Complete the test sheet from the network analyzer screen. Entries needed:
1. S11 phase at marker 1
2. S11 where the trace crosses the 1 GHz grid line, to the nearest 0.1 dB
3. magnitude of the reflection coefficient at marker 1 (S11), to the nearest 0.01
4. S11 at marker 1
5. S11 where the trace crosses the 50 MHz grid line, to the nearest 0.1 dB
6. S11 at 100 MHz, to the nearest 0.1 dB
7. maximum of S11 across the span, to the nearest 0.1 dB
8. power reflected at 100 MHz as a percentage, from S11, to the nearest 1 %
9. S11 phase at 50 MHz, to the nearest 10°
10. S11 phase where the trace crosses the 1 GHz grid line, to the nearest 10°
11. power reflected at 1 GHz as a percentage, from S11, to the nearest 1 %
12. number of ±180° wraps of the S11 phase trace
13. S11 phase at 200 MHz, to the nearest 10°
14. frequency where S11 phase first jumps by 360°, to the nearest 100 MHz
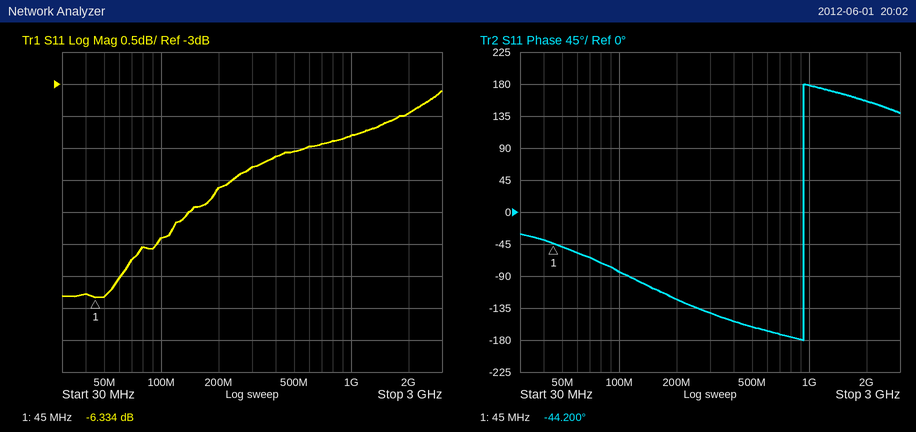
-44.200°
-3.8 dB
0.48
-6.334 dB
-6.3 dB
-5.4 dB
-3.1 dB
29 %
-50°
180°
42 %
1
-120°
900 MHz
